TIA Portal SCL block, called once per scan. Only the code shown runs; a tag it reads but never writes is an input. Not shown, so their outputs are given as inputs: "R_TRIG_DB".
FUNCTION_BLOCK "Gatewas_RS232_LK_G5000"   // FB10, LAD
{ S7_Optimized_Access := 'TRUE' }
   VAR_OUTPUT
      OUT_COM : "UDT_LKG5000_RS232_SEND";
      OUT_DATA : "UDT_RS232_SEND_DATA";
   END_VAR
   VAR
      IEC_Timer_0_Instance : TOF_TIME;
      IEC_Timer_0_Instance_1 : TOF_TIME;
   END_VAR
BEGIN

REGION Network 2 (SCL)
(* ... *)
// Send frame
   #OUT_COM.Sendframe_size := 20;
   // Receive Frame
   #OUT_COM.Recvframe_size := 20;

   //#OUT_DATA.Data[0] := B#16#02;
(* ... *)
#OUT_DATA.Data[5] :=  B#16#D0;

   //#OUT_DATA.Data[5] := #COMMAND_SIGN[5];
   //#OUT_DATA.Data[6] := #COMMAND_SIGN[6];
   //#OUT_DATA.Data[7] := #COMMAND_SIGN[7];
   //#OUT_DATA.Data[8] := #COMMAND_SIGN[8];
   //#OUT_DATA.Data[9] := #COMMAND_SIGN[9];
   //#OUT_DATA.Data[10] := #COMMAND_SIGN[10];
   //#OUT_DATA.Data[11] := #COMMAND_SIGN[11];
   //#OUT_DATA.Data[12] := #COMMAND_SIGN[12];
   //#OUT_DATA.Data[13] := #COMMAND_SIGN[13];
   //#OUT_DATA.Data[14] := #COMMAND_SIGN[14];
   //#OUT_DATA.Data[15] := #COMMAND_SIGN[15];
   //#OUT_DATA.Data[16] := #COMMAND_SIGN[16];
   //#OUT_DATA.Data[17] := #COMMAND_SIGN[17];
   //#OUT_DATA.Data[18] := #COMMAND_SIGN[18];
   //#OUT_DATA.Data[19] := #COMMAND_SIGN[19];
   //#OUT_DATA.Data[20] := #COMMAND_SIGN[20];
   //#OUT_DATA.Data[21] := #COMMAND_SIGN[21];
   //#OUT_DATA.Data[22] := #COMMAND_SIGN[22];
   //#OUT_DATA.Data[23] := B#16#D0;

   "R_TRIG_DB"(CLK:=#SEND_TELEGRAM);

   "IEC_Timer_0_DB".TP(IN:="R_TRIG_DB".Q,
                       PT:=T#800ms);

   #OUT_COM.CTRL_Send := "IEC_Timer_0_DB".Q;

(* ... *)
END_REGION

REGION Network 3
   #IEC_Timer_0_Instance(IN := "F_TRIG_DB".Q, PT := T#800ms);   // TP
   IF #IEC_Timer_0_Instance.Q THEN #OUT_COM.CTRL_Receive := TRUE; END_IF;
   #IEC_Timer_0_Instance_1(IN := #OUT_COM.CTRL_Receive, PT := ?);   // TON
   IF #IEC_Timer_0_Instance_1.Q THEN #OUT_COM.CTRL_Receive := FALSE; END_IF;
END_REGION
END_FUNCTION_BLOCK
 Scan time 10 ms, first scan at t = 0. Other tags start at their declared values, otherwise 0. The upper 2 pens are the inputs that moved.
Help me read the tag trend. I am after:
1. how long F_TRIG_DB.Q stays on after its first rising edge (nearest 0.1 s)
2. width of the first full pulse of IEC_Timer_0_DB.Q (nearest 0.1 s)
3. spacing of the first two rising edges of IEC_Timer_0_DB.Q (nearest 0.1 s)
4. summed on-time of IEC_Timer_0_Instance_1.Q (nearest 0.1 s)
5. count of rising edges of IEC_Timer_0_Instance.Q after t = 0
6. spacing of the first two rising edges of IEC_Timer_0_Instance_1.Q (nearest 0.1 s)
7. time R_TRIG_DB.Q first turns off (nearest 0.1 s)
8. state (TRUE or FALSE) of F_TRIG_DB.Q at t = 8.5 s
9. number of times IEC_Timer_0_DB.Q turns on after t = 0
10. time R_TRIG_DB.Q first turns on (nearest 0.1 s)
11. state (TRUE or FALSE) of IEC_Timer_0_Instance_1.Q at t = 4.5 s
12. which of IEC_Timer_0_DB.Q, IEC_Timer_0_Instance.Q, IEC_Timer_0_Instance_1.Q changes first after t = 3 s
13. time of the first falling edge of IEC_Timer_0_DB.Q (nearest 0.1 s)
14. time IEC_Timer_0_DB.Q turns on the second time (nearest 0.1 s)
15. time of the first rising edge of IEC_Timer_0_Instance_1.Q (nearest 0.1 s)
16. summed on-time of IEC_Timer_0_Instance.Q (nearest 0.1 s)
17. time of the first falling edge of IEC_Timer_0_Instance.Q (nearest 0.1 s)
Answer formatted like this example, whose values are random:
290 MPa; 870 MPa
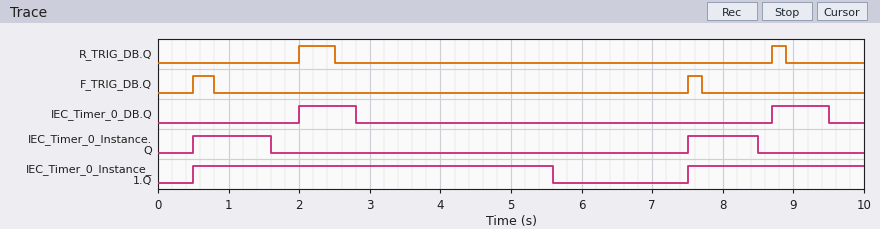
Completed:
0.3 s; 0.8 s; 6.7 s; 7.6 s; 2; 7.0 s; 2.5 s; FALSE; 2; 2.0 s; TRUE; IEC_Timer_0_Instance_1.Q; 2.8 s; 8.7 s; 0.5 s; 2.1 s; 1.6 s
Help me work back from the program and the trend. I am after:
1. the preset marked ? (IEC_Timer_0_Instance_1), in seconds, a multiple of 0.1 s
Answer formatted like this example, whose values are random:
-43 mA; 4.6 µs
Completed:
4.0 s
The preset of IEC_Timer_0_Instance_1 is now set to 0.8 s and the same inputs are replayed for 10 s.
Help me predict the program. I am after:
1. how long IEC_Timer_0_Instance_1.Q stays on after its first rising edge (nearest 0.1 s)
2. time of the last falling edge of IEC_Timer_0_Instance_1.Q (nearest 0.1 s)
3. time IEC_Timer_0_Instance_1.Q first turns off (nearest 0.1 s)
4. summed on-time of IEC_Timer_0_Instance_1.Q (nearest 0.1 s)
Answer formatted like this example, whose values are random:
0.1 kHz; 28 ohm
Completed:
1.9 s; 9.3 s; 2.4 s; 3.7 s
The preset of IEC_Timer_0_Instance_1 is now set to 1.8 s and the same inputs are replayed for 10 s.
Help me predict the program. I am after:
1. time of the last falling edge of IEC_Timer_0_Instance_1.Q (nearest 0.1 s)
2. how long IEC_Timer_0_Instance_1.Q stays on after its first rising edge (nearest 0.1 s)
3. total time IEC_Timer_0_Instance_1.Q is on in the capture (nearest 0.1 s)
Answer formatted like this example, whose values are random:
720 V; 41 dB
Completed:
3.4 s; 2.9 s; 5.4 s
